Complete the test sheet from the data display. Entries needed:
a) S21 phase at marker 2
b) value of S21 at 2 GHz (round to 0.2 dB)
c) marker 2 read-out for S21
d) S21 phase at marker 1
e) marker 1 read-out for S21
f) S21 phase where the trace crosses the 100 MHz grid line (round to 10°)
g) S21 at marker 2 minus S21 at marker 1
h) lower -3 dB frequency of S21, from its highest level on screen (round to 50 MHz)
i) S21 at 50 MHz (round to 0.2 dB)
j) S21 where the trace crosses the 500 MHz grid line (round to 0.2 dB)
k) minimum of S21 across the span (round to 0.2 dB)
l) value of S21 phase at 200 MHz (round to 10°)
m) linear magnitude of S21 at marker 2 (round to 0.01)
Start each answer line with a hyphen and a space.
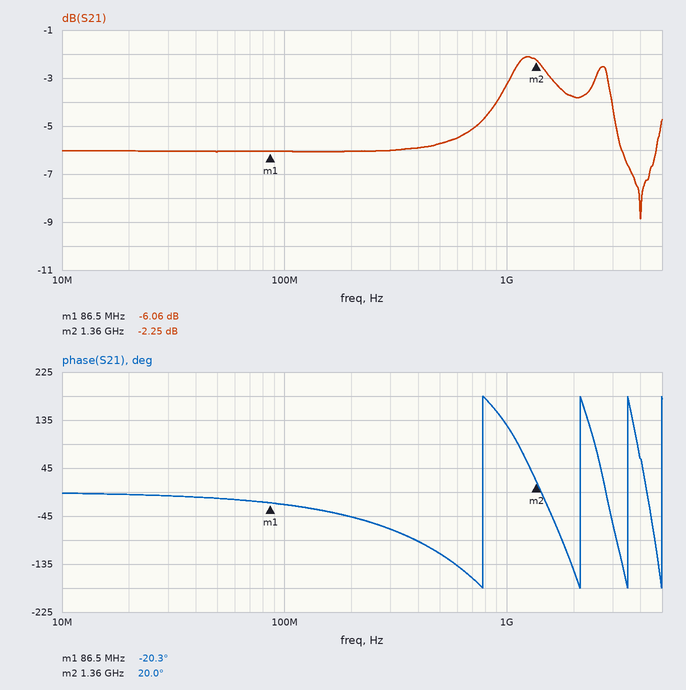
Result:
- 20.0°
- -3.8 dB
- -2.25 dB
- -20.3°
- -6.06 dB
- -20°
- 3.81 dB
- 700 MHz
- -6.0 dB
- -5.8 dB
- -8.8 dB
- -50°
- 0.77
